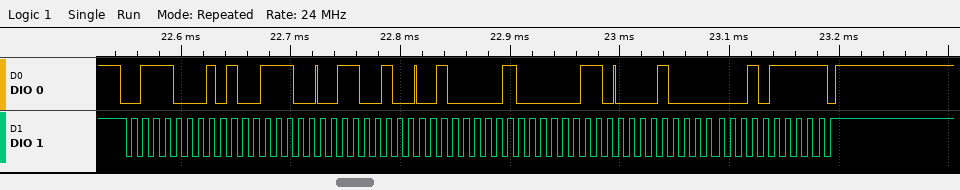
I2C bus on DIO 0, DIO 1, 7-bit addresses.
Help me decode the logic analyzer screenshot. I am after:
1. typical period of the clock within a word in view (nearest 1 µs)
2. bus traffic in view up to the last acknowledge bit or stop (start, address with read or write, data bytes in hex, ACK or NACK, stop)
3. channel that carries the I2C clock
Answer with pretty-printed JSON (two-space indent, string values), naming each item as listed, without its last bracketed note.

{
  "typical period of the clock within a word in view": "10 µs",
  "bus traffic in view up to the last acknowledge bit or stop": "start, address 38 read ACK, 9C ACK, 64 ACK, 41 ACK, 06 ACK, 10 ACK, 2F NACK, stop",
  "channel that carries the I2C clock": "DIO 1"
}
